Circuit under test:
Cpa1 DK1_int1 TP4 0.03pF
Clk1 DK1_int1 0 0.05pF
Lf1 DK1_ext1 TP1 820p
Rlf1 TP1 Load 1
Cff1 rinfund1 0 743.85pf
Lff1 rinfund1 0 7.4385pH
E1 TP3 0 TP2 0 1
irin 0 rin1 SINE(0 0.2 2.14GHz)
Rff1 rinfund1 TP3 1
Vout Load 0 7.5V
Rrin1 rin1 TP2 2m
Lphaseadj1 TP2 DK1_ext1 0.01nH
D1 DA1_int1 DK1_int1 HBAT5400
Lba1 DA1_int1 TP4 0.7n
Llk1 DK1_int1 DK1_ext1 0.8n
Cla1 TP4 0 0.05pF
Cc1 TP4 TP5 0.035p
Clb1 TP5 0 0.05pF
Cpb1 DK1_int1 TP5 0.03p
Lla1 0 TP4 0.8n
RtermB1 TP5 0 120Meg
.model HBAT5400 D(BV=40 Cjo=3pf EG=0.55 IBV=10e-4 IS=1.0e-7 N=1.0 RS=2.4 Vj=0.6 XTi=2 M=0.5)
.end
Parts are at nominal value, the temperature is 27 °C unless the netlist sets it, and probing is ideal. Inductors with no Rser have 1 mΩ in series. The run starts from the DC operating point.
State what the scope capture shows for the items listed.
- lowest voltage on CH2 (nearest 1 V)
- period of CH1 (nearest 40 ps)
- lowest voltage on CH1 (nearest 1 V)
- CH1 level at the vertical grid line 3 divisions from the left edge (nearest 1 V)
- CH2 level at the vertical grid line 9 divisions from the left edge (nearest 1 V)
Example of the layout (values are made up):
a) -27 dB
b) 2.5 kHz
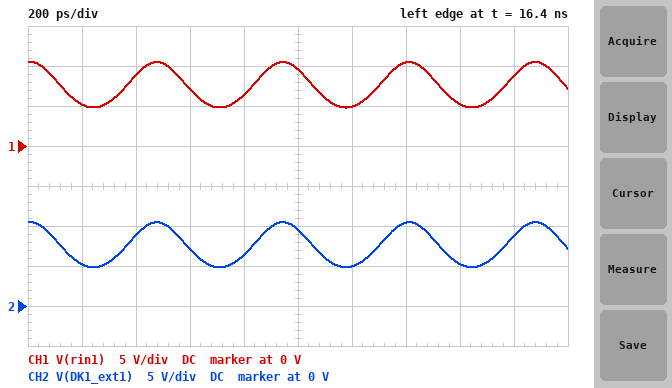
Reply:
a) 5 V
b) 480 ps
c) 5 V
d) 7 V
e) 9 V
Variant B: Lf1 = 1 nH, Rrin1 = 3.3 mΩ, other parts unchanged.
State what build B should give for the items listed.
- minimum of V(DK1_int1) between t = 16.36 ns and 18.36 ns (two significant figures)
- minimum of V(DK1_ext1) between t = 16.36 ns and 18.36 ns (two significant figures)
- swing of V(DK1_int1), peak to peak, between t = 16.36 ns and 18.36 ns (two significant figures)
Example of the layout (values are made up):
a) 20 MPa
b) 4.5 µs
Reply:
a) 3.6 V
b) 4.1 V
c) 8.9 V
